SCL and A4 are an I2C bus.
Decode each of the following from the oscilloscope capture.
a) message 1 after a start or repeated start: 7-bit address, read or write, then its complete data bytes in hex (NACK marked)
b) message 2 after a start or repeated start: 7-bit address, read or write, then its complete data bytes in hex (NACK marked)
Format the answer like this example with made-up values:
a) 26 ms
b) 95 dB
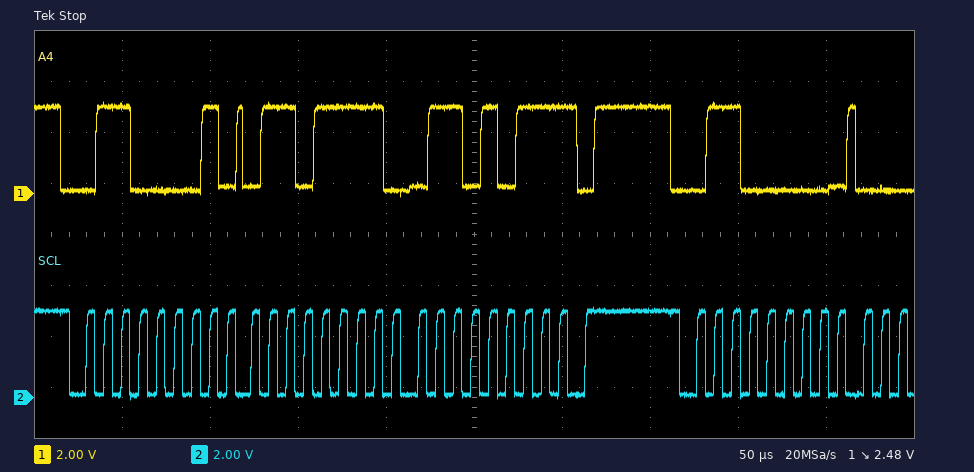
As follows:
a) 0x30 read: 6F 6B NACK
b) 0x30 write
